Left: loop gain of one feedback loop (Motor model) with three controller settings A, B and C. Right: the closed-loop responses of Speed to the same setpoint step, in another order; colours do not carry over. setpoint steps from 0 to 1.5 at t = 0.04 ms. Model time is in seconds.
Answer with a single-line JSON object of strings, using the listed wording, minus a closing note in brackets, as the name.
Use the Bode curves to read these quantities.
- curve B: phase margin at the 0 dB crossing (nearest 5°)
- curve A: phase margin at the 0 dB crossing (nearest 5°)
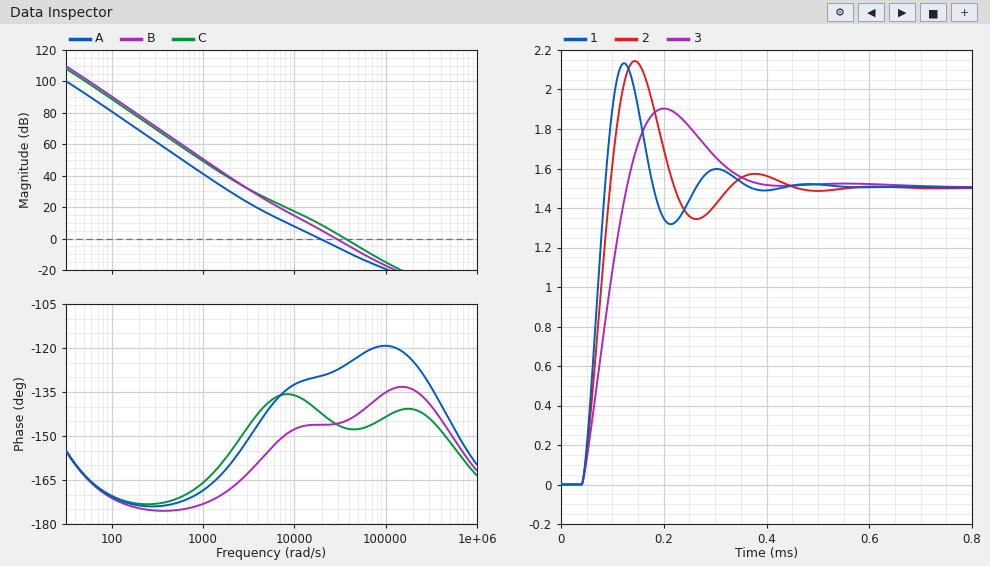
{"curve B: phase margin at the 0 dB crossing": "35°", "curve A: phase margin at the 0 dB crossing": "50°"}
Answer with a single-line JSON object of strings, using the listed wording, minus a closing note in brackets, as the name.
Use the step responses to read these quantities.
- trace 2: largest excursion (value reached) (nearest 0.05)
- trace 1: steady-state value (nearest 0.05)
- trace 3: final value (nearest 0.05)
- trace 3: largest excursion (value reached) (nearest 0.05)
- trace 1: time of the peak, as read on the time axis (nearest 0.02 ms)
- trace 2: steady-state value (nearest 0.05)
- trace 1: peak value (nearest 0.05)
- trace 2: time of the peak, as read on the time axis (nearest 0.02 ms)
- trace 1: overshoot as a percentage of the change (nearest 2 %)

{"trace 2: largest excursion (value reached)": "2.15", "trace 1: steady-state value": "1.50", "trace 3: final value": "1.50", "trace 3: largest excursion (value reached)": "1.90", "trace 1: time of the peak, as read on the time axis": "0.12 ms", "trace 2: steady-state value": "1.50", "trace 1: peak value": "2.15", "trace 2: time of the peak, as read on the time axis": "0.14 ms", "trace 1: overshoot as a percentage of the change": "42 %"}
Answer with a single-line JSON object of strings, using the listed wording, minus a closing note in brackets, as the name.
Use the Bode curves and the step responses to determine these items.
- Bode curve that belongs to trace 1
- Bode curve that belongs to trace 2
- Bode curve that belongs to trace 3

{"Bode curve that belongs to trace 1": "C", "Bode curve that belongs to trace 2": "B", "Bode curve that belongs to trace 3": "A"}
